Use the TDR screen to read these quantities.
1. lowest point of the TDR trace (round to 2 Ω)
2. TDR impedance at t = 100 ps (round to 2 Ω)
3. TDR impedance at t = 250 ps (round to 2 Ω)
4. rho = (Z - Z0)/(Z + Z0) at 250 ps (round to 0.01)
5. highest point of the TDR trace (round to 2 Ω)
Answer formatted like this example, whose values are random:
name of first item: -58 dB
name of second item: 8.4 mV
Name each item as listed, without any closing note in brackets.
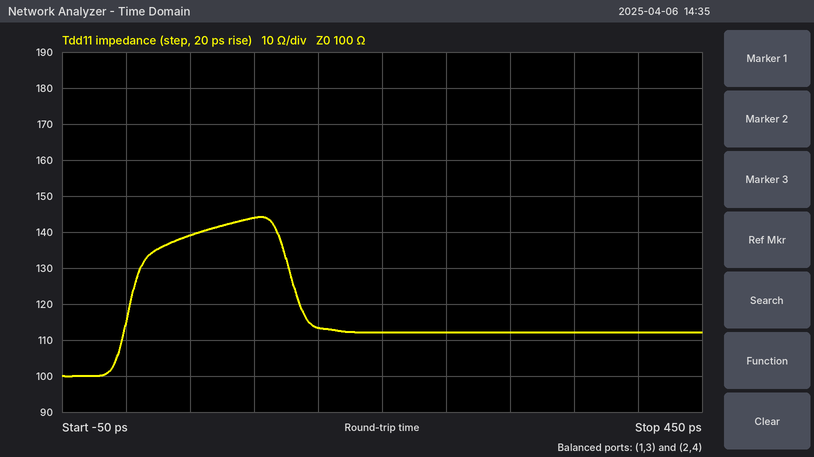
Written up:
lowest point of the TDR trace: 100 Ω
TDR impedance at t = 100 ps: 144 Ω
TDR impedance at t = 250 ps: 112 Ω
rho = (Z - Z0)/(Z + Z0) at 250 ps: +0.06
highest point of the TDR trace: 144 Ω
